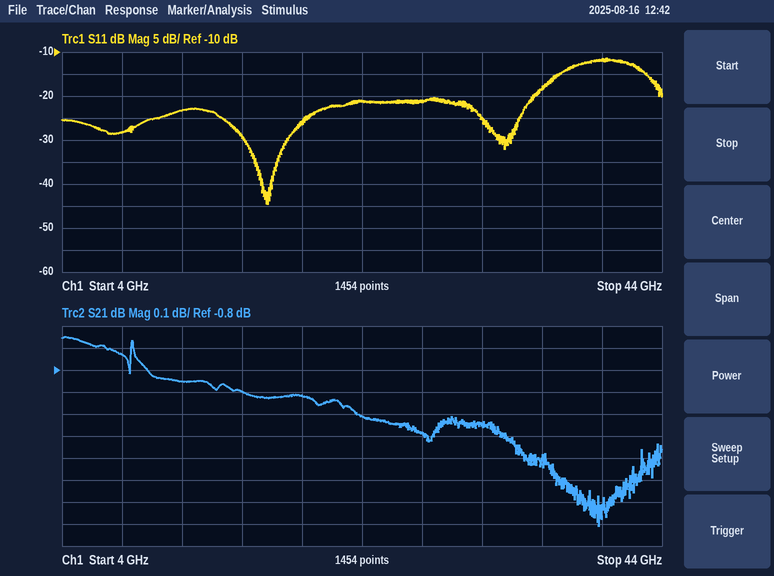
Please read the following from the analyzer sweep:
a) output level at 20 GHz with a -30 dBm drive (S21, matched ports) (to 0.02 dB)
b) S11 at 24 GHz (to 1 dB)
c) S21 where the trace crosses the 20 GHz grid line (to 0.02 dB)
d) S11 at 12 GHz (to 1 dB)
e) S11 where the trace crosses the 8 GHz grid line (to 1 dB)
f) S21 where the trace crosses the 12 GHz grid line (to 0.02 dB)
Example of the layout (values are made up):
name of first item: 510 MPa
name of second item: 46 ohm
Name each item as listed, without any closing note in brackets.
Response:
output level at 20 GHz with a -30 dBm drive (S21, matched ports): -30.92 dBm
S11 at 24 GHz: -21 dB
S21 where the trace crosses the 20 GHz grid line: -0.92 dB
S11 at 12 GHz: -23 dB
S11 where the trace crosses the 8 GHz grid line: -28 dB
S21 where the trace crosses the 12 GHz grid line: -0.86 dB
